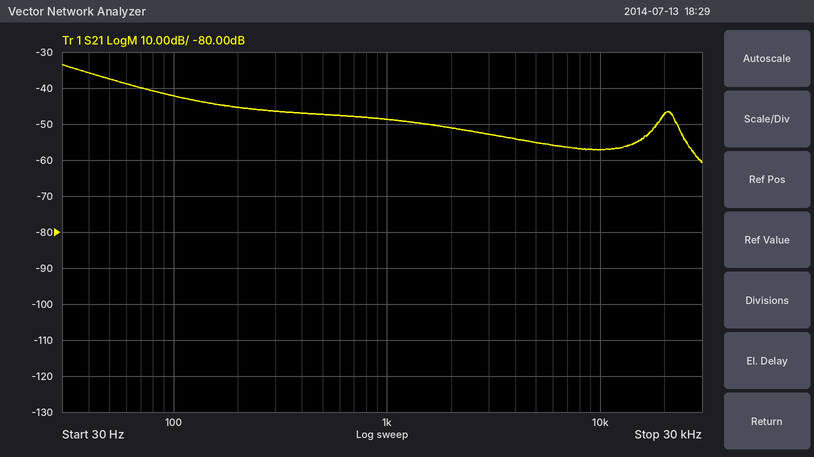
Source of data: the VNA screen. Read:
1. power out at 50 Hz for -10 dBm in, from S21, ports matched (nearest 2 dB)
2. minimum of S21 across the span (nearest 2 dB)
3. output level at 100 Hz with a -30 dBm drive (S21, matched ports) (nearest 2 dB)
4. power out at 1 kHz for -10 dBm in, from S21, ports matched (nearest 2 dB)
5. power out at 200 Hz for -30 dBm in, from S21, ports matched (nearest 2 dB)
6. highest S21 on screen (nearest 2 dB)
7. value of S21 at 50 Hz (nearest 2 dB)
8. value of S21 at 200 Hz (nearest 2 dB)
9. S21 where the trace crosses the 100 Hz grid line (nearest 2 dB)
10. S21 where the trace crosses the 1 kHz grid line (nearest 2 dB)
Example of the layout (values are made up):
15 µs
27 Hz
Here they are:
-48 dBm
-60 dB
-72 dBm
-58 dBm
-76 dBm
-34 dB
-38 dB
-46 dB
-42 dB
-48 dB
